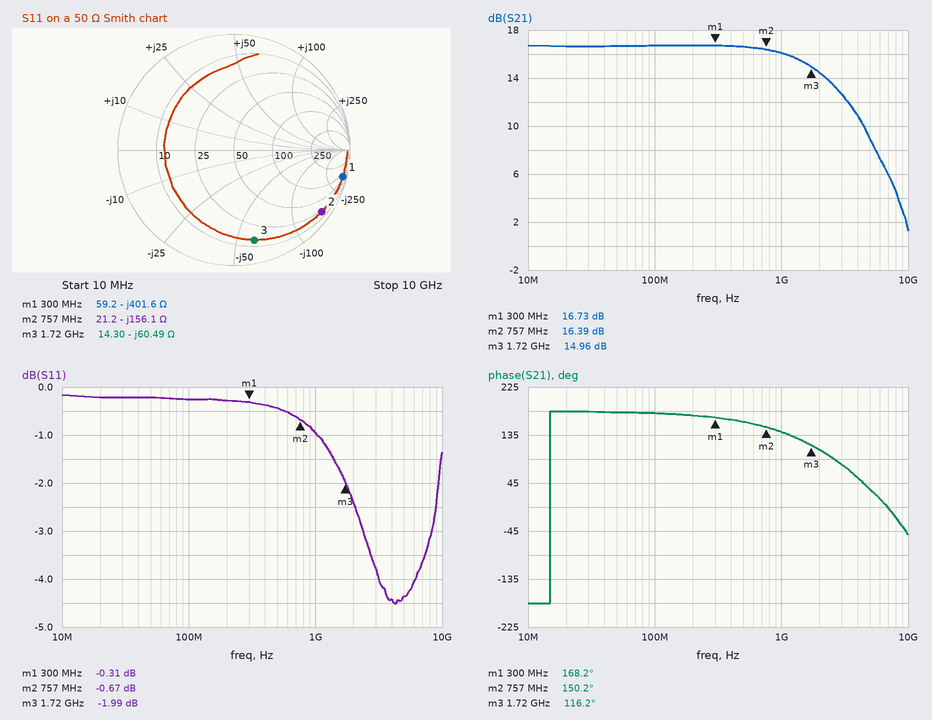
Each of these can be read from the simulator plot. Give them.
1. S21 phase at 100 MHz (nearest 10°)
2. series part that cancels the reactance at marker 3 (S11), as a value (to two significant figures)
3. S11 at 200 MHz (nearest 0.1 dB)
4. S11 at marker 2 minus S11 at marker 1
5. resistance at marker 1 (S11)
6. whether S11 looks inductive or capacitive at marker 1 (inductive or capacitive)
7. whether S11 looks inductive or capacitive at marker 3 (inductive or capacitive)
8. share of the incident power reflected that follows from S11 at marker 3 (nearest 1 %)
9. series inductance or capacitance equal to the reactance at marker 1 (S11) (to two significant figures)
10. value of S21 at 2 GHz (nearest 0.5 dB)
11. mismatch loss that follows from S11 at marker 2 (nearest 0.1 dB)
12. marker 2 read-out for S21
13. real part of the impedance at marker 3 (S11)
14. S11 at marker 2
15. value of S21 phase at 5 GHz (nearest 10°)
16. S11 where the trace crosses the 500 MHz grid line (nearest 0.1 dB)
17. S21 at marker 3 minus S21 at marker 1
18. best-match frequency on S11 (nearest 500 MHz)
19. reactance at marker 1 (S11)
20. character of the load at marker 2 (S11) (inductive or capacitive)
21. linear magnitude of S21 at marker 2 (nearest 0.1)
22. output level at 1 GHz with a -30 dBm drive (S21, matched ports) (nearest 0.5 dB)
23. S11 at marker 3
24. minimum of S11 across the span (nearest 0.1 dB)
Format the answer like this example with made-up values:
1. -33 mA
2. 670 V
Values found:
1. 180°
2. 5.6 nH
3. -0.3 dB
4. -0.36 dB
5. 59.2 Ω
6. capacitive
7. capacitive
8. 63 %
9. 1.3 pF
10. 14.5 dB
11. 8.4 dB
12. 16.39 dB
13. 14.30 Ω
14. -0.67 dB
15. 30°
16. -0.4 dB
17. -1.77 dB
18. 4.5 GHz
19. -401.6 Ω
20. capacitive
21. 6.6
22. -14.0 dBm
23. -1.99 dB
24. -4.5 dB
